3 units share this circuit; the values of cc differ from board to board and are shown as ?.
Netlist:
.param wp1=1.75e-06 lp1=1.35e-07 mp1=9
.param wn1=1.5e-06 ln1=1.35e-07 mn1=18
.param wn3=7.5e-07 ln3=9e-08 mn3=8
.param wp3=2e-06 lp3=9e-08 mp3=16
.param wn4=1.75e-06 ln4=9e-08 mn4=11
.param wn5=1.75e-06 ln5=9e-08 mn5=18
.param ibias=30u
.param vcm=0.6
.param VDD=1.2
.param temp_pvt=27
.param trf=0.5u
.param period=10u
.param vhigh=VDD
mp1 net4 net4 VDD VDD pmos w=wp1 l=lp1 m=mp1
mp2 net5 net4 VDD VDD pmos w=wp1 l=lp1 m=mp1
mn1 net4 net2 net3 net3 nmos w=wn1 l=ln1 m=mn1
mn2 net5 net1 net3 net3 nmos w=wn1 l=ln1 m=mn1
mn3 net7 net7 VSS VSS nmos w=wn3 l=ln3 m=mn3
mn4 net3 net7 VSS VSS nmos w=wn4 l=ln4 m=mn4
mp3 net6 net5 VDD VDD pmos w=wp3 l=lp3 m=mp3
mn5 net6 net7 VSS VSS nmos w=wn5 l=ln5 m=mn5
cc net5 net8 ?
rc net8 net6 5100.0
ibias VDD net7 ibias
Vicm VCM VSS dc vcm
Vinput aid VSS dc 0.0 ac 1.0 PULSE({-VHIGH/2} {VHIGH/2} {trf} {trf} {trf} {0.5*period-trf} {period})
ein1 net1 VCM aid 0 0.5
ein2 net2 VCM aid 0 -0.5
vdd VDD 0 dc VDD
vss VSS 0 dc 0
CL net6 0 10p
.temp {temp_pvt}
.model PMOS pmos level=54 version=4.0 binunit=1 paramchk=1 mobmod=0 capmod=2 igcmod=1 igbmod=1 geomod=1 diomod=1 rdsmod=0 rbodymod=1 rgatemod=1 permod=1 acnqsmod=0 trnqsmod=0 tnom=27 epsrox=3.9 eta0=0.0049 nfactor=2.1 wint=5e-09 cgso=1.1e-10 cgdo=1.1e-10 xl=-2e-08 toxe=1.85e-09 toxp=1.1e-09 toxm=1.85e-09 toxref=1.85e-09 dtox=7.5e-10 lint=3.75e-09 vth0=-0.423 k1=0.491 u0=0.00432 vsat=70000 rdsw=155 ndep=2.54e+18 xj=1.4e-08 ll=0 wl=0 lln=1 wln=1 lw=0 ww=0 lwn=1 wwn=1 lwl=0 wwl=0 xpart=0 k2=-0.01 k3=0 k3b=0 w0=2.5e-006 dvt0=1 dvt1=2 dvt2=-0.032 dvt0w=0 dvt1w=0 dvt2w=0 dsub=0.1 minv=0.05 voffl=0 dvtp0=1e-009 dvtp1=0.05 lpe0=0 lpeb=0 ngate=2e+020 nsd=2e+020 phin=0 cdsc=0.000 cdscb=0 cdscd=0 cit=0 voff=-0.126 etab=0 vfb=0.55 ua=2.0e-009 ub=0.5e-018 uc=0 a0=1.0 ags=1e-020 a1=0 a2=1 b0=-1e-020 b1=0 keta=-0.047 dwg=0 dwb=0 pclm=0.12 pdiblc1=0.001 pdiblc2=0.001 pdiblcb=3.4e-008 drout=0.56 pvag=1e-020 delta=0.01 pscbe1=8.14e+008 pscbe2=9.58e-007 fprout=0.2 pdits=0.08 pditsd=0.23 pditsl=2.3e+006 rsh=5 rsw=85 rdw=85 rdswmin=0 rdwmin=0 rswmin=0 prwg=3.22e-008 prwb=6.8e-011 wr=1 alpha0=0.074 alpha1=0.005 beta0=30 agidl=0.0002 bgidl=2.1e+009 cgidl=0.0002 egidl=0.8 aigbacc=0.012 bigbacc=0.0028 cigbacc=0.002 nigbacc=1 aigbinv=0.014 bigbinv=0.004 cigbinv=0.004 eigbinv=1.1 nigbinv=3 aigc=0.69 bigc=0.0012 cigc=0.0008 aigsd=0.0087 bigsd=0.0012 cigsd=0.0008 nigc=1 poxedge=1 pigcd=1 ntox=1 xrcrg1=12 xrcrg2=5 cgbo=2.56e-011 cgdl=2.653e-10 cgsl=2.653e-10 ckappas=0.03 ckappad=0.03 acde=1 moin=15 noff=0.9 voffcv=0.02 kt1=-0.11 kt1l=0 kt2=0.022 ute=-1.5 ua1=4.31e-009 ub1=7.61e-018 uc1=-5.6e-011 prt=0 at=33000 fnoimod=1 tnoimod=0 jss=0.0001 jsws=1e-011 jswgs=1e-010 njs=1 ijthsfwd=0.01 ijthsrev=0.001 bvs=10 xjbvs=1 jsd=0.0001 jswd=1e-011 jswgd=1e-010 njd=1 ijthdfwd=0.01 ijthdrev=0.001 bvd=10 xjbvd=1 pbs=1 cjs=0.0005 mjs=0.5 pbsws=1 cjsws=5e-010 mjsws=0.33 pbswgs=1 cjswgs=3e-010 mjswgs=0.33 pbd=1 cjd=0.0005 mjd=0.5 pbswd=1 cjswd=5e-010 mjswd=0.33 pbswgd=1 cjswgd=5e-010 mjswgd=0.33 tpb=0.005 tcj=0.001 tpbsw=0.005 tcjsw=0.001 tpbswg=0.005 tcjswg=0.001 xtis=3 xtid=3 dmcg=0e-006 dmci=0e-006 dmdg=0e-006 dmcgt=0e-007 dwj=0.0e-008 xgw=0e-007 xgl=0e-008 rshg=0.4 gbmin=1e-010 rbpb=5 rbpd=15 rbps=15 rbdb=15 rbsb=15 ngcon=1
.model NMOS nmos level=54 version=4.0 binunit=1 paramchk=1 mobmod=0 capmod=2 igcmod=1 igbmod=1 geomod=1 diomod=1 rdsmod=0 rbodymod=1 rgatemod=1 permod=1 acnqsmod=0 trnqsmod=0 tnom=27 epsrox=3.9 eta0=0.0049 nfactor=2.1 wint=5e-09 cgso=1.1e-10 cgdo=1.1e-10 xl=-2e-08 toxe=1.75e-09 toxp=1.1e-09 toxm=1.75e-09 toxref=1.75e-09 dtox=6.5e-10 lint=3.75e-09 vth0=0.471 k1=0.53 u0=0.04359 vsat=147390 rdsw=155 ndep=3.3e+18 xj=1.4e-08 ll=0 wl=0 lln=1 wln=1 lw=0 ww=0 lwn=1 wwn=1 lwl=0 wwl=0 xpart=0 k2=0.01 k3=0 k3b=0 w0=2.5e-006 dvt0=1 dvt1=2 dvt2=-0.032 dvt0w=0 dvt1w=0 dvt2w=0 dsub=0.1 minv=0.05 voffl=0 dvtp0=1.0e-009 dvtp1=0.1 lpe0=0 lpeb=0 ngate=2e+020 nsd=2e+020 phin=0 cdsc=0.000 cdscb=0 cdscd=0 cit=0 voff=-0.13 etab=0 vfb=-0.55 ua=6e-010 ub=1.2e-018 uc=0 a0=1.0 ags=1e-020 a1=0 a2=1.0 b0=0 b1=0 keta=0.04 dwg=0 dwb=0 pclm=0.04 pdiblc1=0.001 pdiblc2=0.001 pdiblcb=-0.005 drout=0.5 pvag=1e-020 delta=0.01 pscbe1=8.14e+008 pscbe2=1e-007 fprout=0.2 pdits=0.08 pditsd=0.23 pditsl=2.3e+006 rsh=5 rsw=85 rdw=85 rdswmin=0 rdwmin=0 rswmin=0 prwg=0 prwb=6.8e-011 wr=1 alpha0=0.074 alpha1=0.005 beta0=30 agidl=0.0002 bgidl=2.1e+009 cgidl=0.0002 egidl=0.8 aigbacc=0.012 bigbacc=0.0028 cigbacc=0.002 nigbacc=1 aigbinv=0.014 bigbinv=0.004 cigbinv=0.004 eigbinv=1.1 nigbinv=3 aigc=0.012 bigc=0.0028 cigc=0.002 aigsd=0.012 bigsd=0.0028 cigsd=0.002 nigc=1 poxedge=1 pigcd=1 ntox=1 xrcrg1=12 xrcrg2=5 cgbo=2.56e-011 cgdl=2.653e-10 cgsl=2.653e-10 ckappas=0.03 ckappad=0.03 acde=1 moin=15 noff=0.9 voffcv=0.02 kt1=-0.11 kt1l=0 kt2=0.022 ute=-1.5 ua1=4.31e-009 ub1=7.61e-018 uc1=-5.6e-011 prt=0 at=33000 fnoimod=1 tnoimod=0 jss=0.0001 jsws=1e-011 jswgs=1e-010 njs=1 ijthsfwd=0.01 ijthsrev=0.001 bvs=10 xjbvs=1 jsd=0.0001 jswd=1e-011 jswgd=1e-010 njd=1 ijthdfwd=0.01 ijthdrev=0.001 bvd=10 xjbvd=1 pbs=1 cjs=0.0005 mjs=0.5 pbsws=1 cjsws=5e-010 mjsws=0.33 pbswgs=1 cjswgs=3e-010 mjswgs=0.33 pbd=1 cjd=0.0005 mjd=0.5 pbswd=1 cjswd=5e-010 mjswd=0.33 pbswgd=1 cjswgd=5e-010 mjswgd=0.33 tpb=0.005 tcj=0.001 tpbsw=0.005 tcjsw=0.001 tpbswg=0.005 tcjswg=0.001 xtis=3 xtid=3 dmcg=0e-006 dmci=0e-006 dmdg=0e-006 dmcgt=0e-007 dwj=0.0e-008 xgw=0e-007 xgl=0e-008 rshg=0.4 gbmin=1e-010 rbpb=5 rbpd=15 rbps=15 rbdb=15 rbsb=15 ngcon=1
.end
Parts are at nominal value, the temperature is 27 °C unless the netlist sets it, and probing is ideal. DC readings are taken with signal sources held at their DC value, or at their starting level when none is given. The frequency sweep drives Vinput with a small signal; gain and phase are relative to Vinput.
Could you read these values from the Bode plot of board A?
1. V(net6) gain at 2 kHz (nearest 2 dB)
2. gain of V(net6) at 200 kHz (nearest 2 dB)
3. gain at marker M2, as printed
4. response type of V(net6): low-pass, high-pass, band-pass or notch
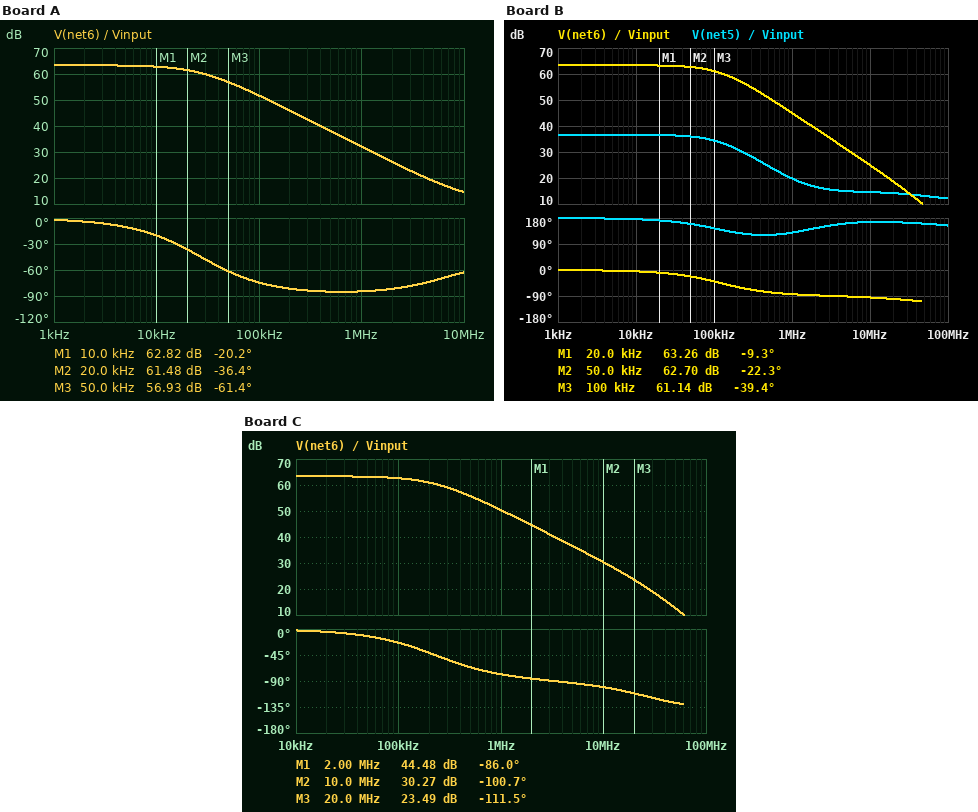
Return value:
64 dB
46 dB
61.48 dB
low-pass
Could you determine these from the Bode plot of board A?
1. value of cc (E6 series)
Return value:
3.3 pF
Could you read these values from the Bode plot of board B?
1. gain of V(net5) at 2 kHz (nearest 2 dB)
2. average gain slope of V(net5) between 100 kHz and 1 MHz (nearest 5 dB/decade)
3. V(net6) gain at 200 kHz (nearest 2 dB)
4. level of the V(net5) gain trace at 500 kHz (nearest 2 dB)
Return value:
36 dB
-15 dB/decade
58 dB
24 dB
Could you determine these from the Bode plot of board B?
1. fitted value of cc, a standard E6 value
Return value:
680 fF
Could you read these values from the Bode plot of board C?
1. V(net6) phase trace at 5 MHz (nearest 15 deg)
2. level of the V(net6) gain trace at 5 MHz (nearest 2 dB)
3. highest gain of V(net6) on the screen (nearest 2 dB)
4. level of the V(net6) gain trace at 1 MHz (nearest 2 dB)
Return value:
-90 deg
36 dB
64 dB
50 dB
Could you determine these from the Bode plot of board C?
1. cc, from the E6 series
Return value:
330 fF
